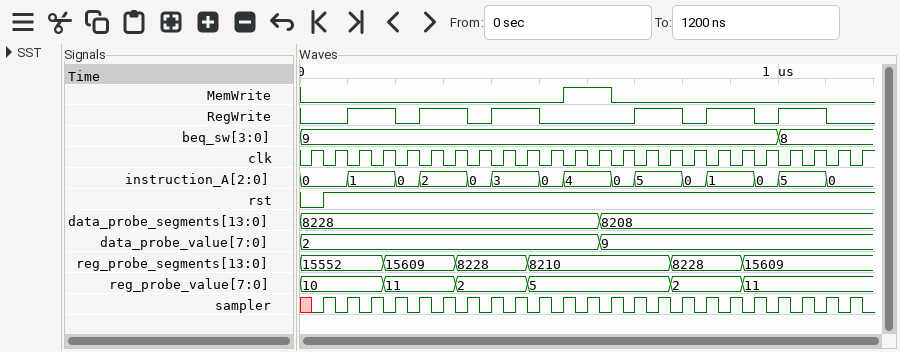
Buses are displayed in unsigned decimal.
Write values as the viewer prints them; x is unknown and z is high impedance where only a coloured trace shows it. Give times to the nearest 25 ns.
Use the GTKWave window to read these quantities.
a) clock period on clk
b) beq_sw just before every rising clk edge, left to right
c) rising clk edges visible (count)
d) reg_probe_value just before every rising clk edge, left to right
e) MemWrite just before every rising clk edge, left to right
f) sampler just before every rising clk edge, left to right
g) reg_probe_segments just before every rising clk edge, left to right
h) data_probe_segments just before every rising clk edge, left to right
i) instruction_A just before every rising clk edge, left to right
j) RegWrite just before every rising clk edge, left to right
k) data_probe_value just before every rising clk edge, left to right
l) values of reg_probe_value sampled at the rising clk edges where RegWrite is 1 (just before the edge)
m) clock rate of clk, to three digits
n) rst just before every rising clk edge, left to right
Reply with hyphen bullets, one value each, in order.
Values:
- 50 ns
- 9, 9, 9, 9, 9, 9, 9, 9, 9, 9, 9, 9, 9, 9, 9, 9, 9, 9, 9, 9, 8, 8, 8, 8
- 24
- 10, 10, 10, 10, 11, 11, 11, 2, 2, 2, 5, 5, 5, 5, 5, 5, 2, 2, 2, 11, 11, 11, 11, 11
- 0 0 0 0 0 0 0 0 0 0 0 1 1 0 0 0 0 0 0 0 0 0 0 0
- x 1 1 1 1 1 1 1 1 1 1 1 1 1 1 1 1 1 1 1 1 1 1 1
- 15552, 15552, 15552, 15552, 15609, 15609, 15609, 8228, 8228, 8228, 8210, 8210, 8210, 8210, 8210, 8210, 8228, 8228, 8228, 15609, 15609, 15609, 15609, 15609
- 8228, 8228, 8228, 8228, 8228, 8228, 8228, 8228, 8228, 8228, 8228, 8228, 8228, 8208, 8208, 8208, 8208, 8208, 8208, 8208, 8208, 8208, 8208, 8208
- 0, 0, 1, 1, 0, 2, 2, 0, 3, 3, 0, 4, 4, 0, 5, 5, 0, 1, 1, 0, 5, 5, 0, 0
- 0 0 1 1 0 1 1 0 1 1 0 0 0 0 1 1 0 1 1 0 1 1 0 0
- 2, 2, 2, 2, 2, 2, 2, 2, 2, 2, 2, 2, 2, 9, 9, 9, 9, 9, 9, 9, 9, 9, 9, 9
- 10, 10, 11, 11, 2, 2, 5, 5, 2, 2, 11, 11
- 20.0 MHz
- 0 1 1 1 1 1 1 1 1 1 1 1 1 1 1 1 1 1 1 1 1 1 1 1
